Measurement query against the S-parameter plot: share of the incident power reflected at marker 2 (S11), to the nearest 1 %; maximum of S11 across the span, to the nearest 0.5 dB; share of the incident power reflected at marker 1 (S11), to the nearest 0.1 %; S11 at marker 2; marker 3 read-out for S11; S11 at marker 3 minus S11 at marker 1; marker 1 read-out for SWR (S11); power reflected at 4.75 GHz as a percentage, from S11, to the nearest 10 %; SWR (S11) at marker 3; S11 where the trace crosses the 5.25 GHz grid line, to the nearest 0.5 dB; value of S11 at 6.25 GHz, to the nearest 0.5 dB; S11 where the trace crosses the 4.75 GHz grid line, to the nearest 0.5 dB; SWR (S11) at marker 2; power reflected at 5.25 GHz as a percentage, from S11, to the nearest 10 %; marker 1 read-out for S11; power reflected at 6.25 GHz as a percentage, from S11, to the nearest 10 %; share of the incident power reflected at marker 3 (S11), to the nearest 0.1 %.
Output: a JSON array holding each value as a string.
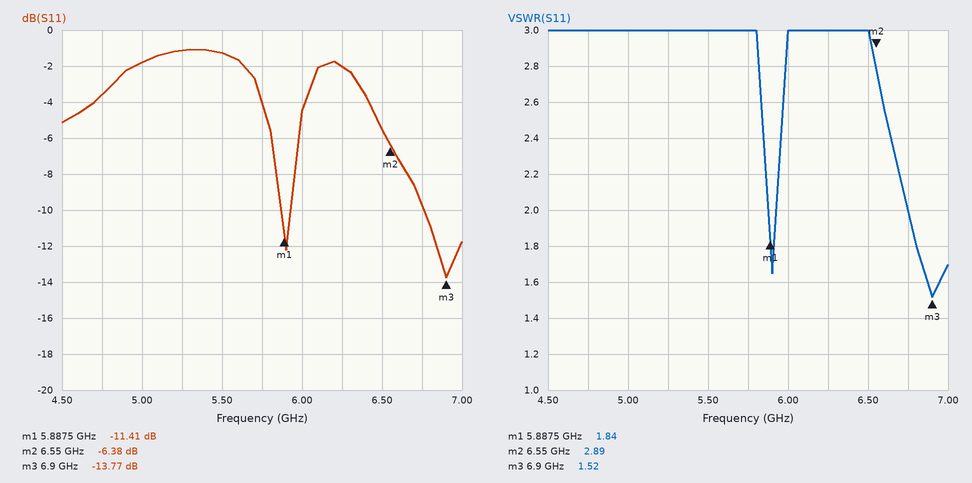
["23 %", "-1.0 dB", "7.2 %", "-6.38 dB", "-13.77 dB", "-2.36 dB", "1.84", "40 %", "1.52", "-1.0 dB", "-2.0 dB", "-3.5 dB", "2.89", "80 %", "-11.41 dB", "60 %", "4.2 %"]
